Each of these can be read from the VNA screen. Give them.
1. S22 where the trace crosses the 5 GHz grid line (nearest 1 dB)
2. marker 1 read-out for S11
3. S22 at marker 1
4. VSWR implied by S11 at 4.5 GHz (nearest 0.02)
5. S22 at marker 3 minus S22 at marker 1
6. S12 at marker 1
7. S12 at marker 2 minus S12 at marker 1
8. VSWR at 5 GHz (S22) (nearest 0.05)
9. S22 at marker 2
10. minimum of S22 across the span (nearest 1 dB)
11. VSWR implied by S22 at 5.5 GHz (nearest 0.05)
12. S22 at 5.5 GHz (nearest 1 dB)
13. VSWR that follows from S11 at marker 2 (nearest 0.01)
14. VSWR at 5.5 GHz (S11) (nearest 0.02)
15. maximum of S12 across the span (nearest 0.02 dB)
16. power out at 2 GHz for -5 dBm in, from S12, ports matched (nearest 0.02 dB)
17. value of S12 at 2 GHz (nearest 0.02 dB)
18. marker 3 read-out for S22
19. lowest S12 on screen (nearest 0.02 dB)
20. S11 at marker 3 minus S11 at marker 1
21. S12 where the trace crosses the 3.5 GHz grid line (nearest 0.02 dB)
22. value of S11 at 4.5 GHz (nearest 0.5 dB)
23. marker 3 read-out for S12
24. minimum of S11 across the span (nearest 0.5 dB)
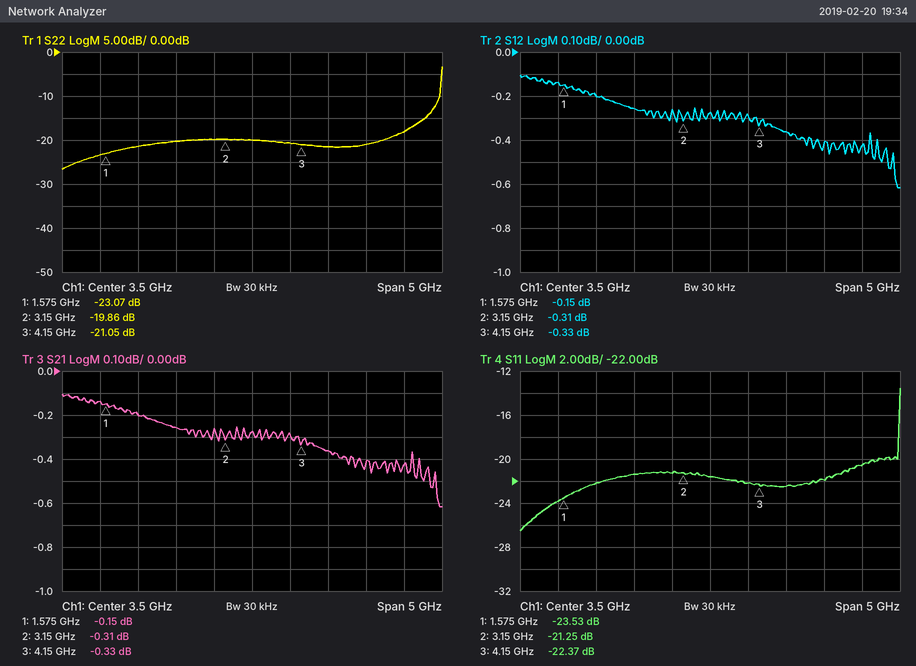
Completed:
-21 dB
-23.53 dB
-23.07 dB
1.16
2.02 dB
-0.15 dB
-0.16 dB
1.20
-19.86 dB
-27 dB
1.30
-18 dB
1.19
1.20
-0.10 dB
-5.20 dBm
-0.20 dB
-21.05 dB
-0.62 dB
1.16 dB
-0.28 dB
-22.5 dB
-0.33 dB
-26.5 dB
